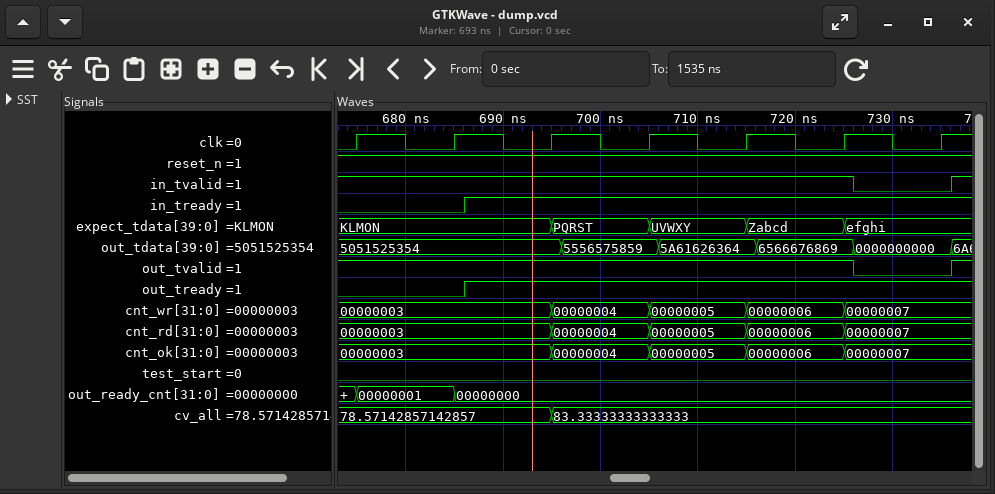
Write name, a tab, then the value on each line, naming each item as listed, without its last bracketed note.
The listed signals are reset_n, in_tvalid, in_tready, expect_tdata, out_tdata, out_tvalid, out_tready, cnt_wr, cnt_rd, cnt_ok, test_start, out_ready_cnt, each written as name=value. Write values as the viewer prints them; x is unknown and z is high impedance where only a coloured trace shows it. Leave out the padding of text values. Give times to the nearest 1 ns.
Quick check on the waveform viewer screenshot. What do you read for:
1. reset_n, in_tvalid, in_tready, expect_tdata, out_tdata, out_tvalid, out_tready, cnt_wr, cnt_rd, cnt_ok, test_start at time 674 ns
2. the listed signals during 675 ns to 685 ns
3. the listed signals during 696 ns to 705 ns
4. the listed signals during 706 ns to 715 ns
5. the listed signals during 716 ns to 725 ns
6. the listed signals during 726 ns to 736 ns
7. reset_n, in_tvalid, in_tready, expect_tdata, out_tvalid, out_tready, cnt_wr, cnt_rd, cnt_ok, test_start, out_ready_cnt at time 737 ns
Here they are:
reset_n, in_tvalid, in_tready, expect_tdata, out_tdata, out_tvalid, out_tready, cnt_wr, cnt_rd, cnt_ok, test_start at time 674 ns	reset_n=1, in_tvalid=1, in_tready=0, expect_tdata=KLMON, out_tdata=5051525354, out_tvalid=1, out_tready=0, cnt_wr=00000003, cnt_rd=00000003, cnt_ok=00000003, test_start=0
the listed signals during 675 ns to 685 ns	reset_n=1, in_tvalid=1, in_tready=0, expect_tdata=KLMON, out_tdata=5051525354, out_tvalid=1, out_tready=0, cnt_wr=00000003, cnt_rd=00000003, cnt_ok=00000003, test_start=0, out_ready_cnt=00000001
the listed signals during 696 ns to 705 ns	reset_n=1, in_tvalid=1, in_tready=1, expect_tdata=PQRST, out_tdata=5556575859, out_tvalid=1, out_tready=1, cnt_wr=00000004, cnt_rd=00000004, cnt_ok=00000004, test_start=0, out_ready_cnt=00000000
the listed signals during 706 ns to 715 ns	reset_n=1, in_tvalid=1, in_tready=1, expect_tdata=UVWXY, out_tdata=5A61626364, out_tvalid=1, out_tready=1, cnt_wr=00000005, cnt_rd=00000005, cnt_ok=00000005, test_start=0, out_ready_cnt=00000000
the listed signals during 716 ns to 725 ns	reset_n=1, in_tvalid=1, in_tready=1, expect_tdata=Zabcd, out_tdata=6566676869, out_tvalid=1, out_tready=1, cnt_wr=00000006, cnt_rd=00000006, cnt_ok=00000006, test_start=0, out_ready_cnt=00000000
the listed signals during 726 ns to 736 ns	reset_n=1, in_tvalid=0, in_tready=1, expect_tdata=efghi, out_tdata=0000000000, out_tvalid=0, out_tready=1, cnt_wr=00000007, cnt_rd=00000007, cnt_ok=00000007, test_start=0, out_ready_cnt=00000000
reset_n, in_tvalid, in_tready, expect_tdata, out_tvalid, out_tready, cnt_wr, cnt_rd, cnt_ok, test_start, out_ready_cnt at time 737 ns	reset_n=1, in_tvalid=1, in_tready=1, expect_tdata=efghi, out_tvalid=1, out_tready=1, cnt_wr=00000007, cnt_rd=00000007, cnt_ok=00000007, test_start=0, out_ready_cnt=00000000
